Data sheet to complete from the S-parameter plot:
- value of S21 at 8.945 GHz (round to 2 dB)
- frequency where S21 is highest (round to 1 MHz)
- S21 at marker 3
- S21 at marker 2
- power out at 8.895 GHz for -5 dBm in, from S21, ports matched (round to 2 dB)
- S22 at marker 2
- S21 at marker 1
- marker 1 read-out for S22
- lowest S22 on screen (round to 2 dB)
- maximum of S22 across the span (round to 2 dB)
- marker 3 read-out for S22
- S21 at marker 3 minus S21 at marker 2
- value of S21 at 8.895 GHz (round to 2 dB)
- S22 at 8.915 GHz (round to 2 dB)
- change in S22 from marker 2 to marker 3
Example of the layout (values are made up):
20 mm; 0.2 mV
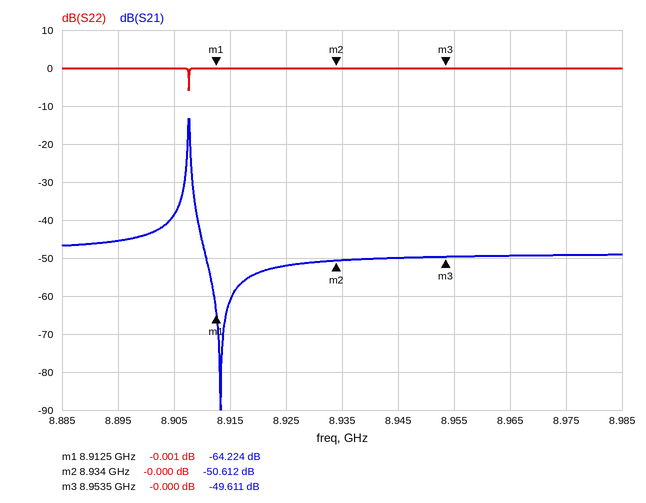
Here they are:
-50 dB; 8.908 GHz; -49.611 dB; -50.612 dB; -50 dBm; -0.000 dB; -64.224 dB; -0.001 dB; -6 dB; 0 dB; -0.000 dB; 1.001 dB; -46 dB; 0 dB; 0.000 dB
